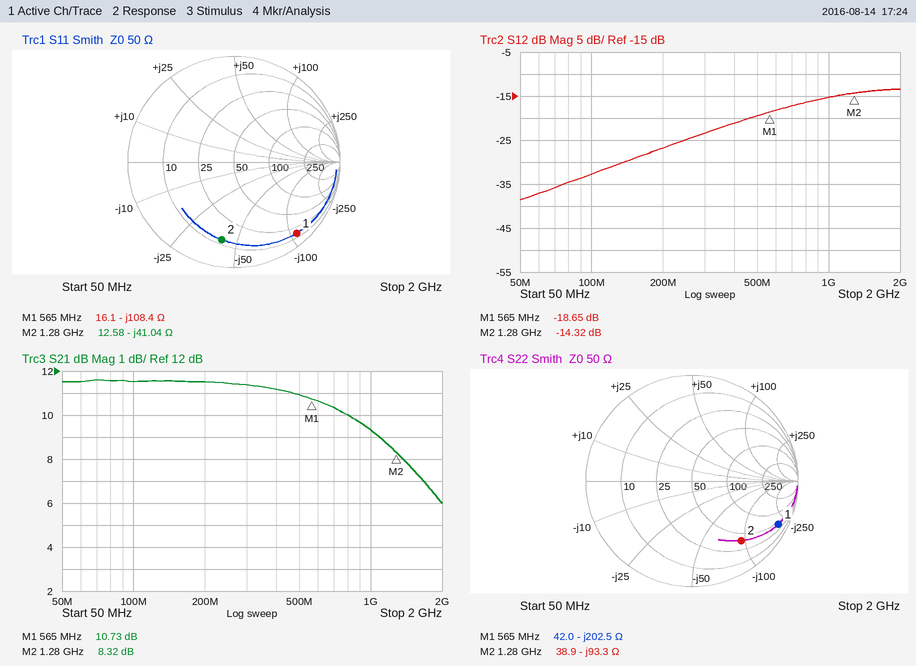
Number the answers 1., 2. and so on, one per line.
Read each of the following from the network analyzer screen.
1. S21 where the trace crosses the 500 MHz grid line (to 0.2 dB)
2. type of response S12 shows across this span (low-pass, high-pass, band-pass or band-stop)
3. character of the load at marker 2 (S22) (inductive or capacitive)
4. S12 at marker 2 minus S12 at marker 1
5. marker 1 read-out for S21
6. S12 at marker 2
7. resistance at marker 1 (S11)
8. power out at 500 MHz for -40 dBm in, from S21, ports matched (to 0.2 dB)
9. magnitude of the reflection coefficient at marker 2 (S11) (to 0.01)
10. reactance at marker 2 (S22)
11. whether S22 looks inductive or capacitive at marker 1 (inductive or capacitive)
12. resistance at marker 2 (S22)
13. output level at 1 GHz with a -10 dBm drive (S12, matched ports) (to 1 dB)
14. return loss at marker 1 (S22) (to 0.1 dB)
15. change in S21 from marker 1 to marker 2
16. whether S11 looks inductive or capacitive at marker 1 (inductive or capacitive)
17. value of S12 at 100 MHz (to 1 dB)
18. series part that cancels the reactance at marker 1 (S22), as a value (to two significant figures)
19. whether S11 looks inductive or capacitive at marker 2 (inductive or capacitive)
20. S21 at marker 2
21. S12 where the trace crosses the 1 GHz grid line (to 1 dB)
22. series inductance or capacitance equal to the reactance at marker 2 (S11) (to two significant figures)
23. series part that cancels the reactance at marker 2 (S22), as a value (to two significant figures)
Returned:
1. 11.0 dB
2. high-pass
3. capacitive
4. 4.33 dB
5. 10.73 dB
6. -14.32 dB
7. 16.1 Ω
8. -29.0 dBm
9. 0.74
10. -93.3 Ω
11. capacitive
12. 38.9 Ω
13. -25 dBm
14. 0.8 dB
15. -2.41 dB
16. capacitive
17. -33 dB
18. 57 nH
19. capacitive
20. 8.32 dB
21. -15 dB
22. 3.0 pF
23. 12 nH
